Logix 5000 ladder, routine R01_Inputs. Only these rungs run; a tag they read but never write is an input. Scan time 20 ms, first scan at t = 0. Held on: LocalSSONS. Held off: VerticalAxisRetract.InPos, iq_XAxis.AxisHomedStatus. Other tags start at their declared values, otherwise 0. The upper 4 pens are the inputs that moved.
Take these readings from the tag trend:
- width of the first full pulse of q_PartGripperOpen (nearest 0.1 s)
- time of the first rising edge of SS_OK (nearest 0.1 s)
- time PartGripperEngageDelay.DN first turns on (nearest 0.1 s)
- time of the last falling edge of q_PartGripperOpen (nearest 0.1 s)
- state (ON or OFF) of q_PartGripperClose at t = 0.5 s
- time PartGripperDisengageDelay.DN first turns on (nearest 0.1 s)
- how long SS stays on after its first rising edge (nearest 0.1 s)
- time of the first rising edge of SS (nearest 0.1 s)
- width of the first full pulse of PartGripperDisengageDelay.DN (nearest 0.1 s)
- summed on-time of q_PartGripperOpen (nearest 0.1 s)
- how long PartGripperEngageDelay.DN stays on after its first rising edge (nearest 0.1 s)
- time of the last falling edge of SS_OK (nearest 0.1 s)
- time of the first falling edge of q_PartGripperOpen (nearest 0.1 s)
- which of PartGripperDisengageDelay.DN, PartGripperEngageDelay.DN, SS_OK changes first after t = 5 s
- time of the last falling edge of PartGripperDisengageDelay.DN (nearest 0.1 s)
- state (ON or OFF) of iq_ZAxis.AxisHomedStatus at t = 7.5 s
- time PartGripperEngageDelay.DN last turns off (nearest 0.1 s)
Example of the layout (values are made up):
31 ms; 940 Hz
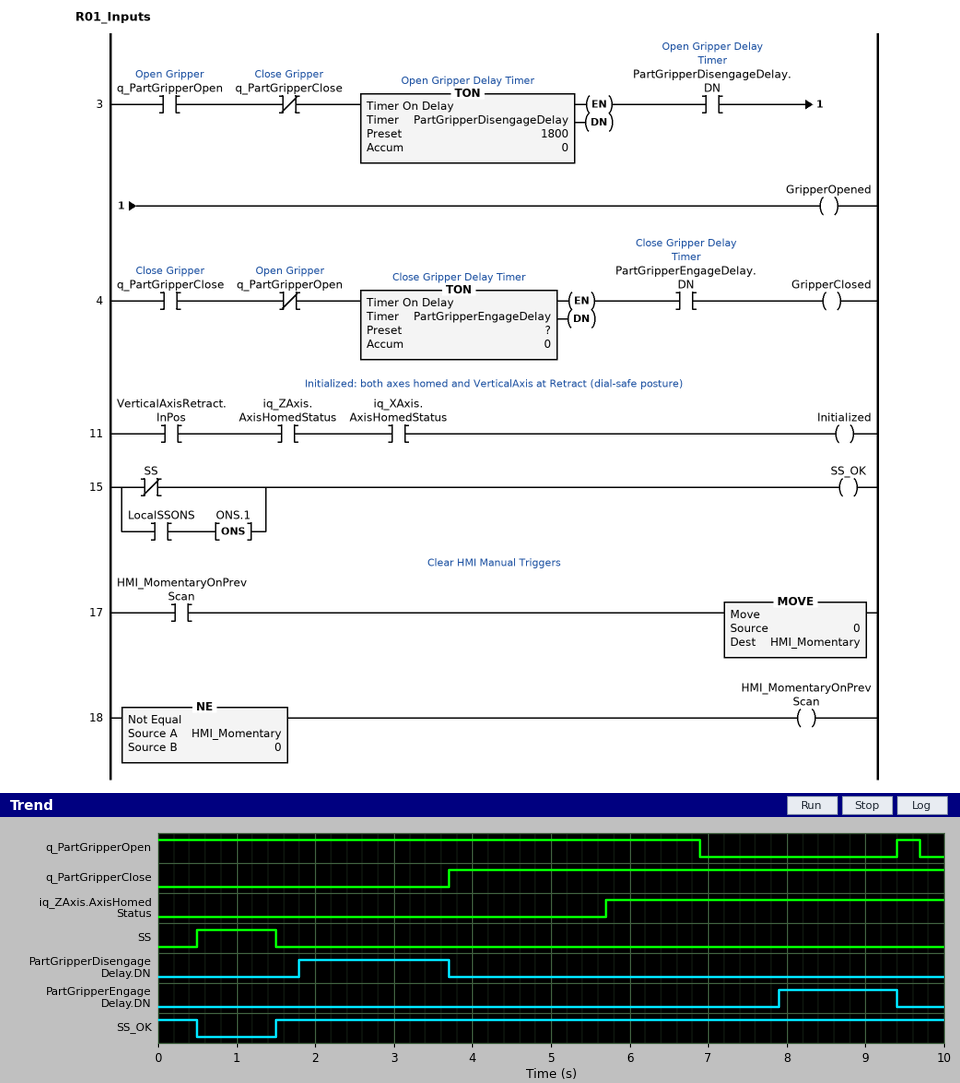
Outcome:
0.3 s; 1.5 s; 7.9 s; 9.7 s; OFF; 1.8 s; 1.0 s; 0.5 s; 1.9 s; 7.2 s; 1.5 s; 0.5 s; 6.9 s; PartGripperEngageDelay.DN; 3.7 s; ON; 9.4 s
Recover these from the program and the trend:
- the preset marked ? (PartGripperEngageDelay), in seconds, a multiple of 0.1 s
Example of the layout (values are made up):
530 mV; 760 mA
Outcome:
1.0 s
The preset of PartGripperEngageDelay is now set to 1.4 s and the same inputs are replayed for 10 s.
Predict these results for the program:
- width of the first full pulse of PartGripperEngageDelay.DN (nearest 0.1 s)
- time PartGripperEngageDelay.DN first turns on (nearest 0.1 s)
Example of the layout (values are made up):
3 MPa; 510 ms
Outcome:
1.1 s; 8.3 s
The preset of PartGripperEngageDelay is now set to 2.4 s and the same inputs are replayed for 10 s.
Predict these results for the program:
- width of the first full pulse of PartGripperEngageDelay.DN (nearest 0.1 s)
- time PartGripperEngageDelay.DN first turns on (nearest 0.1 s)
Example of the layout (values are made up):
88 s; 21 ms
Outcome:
0.1 s; 9.3 s
